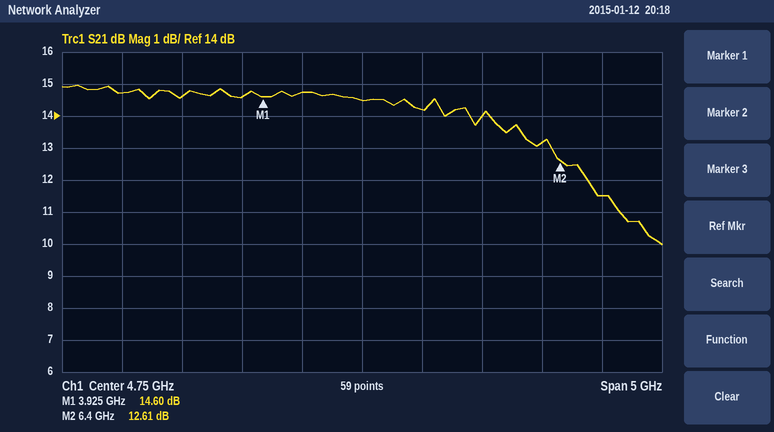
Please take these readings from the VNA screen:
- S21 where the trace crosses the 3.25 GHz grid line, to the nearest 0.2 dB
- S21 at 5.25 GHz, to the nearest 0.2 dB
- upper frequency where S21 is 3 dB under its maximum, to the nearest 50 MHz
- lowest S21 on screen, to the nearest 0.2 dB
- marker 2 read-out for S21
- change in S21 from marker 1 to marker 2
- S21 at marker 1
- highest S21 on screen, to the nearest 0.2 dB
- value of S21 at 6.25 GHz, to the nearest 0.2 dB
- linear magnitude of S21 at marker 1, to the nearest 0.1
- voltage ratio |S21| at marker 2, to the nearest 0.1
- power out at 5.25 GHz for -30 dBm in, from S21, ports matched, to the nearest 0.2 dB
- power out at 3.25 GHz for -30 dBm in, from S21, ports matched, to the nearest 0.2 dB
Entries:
14.6 dB
14.2 dB
6.65 GHz
10.0 dB
12.61 dB
-1.99 dB
14.60 dB
15.0 dB
13.2 dB
5.4
4.3
-15.8 dBm
-15.4 dBm
